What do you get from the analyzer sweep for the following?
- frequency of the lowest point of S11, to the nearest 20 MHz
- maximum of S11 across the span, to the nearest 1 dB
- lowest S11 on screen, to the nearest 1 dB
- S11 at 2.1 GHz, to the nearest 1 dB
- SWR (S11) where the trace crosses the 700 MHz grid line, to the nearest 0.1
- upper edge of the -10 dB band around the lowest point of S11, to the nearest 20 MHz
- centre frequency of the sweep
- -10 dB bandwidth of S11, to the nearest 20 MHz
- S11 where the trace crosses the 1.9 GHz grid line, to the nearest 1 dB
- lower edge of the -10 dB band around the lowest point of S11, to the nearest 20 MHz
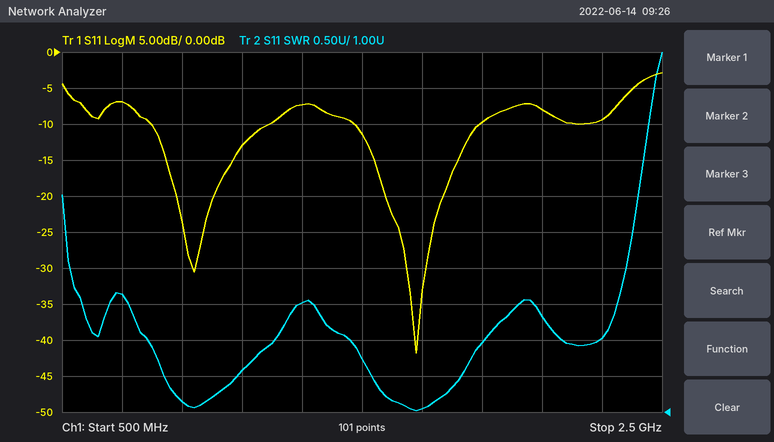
1.68 GHz
-3 dB
-42 dB
-8 dB
2.6
1.90 GHz
1.5 GHz
420 MHz
-10 dB
1.48 GHz
